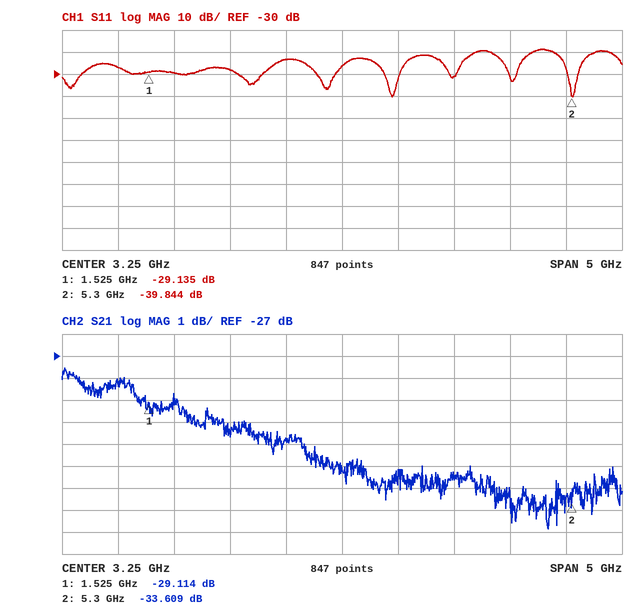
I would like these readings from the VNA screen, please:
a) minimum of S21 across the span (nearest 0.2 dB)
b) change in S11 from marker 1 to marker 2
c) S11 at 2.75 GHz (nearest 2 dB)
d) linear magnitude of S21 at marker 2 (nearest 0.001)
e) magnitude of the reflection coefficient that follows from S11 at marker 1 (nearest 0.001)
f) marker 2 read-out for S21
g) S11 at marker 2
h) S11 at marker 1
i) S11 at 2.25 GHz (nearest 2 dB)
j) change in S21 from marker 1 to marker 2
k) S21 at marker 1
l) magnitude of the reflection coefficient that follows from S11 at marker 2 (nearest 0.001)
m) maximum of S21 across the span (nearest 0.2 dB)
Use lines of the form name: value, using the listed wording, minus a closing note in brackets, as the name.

minimum of S21 across the span: -34.8 dB
change in S11 from marker 1 to marker 2: -10.709 dB
S11 at 2.75 GHz: -24 dB
linear magnitude of S21 at marker 2: 0.021
magnitude of the reflection coefficient that follows from S11 at marker 1: 0.035
marker 2 read-out for S21: -33.609 dB
S11 at marker 2: -39.844 dB
S11 at marker 1: -29.135 dB
S11 at 2.25 GHz: -28 dB
change in S21 from marker 1 to marker 2: -4.495 dB
S21 at marker 1: -29.114 dB
magnitude of the reflection coefficient that follows from S11 at marker 2: 0.010
maximum of S21 across the span: -27.6 dB
